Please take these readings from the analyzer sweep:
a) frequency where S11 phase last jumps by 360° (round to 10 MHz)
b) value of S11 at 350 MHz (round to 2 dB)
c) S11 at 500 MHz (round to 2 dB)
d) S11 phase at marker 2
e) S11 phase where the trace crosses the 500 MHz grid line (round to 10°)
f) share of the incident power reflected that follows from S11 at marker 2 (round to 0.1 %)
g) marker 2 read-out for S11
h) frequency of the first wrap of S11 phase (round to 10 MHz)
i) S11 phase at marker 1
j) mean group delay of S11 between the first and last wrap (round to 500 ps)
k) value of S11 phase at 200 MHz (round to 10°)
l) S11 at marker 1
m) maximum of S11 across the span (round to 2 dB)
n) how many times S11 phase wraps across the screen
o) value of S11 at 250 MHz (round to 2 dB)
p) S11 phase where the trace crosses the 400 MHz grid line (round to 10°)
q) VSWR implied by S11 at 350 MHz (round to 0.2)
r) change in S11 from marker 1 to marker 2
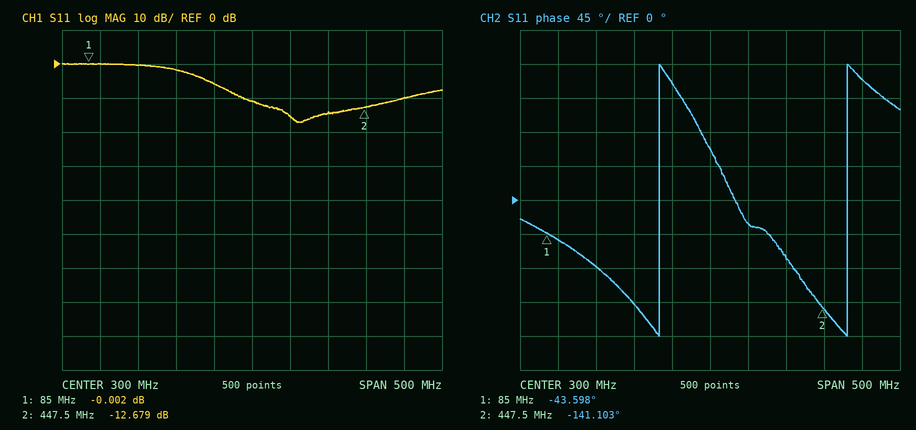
480 MHz
-16 dB
-10 dB
-141.103°
160°
5.4 %
-12.679 dB
230 MHz
-43.598°
4.0 ns
-140°
-0.002 dB
0 dB
2
-6 dB
-80°
1.4
-12.677 dB
